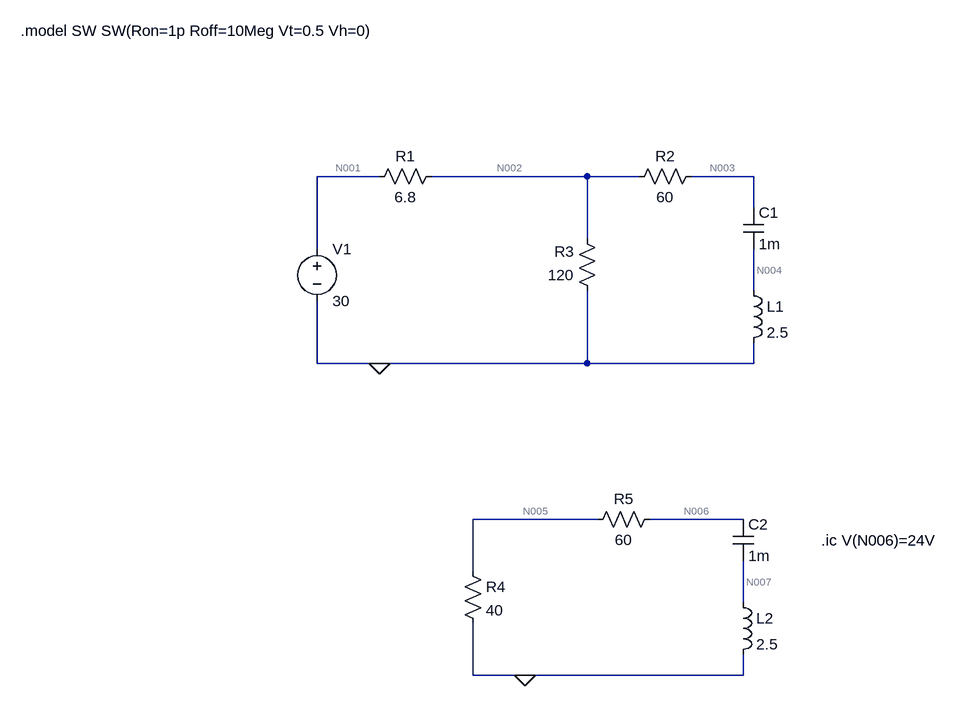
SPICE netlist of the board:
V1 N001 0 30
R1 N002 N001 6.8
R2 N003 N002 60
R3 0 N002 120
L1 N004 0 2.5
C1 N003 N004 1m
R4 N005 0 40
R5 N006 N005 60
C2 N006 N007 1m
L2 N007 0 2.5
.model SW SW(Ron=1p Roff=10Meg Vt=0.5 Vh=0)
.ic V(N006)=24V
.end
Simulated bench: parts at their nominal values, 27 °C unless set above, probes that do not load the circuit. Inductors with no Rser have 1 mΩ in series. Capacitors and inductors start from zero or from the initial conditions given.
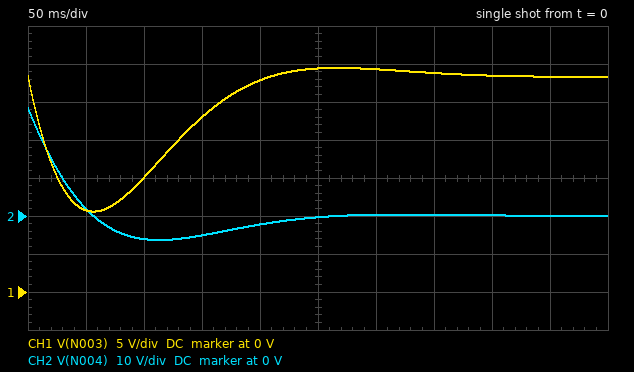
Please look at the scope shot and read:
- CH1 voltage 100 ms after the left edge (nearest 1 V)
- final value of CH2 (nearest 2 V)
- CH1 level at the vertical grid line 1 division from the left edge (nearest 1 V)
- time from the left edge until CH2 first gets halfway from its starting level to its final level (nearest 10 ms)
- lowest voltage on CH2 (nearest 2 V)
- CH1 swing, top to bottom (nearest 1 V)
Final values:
15 V
0 V
11 V
20 ms
-6 V
19 V
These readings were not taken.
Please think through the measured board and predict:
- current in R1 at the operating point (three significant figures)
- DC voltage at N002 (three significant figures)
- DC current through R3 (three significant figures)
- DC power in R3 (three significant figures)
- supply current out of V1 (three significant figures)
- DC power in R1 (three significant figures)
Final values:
237 mA
28.4 V
237 mA
6.72 W
237 mA
381 mW
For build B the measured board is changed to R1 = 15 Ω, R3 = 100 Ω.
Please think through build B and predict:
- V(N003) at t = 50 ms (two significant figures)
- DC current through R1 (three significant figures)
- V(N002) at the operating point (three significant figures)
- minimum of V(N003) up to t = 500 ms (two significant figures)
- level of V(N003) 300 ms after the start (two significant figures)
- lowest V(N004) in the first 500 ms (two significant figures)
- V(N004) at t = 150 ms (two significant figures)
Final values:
9.1 V
261 mA
26.1 V
9.0 V
27 V
-5.2 V
-4.1 V
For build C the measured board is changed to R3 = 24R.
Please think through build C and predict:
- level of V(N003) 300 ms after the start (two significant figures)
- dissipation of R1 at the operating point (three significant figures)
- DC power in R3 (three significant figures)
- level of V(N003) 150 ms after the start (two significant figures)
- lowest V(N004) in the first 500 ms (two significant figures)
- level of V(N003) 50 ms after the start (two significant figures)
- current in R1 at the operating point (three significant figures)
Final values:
24 V
6.45 W
22.8 W
19 V
-5.3 V
9.0 V
974 mA
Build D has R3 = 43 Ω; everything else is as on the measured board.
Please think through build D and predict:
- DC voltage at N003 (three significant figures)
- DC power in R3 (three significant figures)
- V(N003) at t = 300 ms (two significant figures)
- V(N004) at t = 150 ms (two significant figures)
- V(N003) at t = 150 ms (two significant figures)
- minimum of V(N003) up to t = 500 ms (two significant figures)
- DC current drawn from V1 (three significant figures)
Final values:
25.9 V
15.6 W
27 V
-4.7 V
21 V
9.7 V
602 mA
